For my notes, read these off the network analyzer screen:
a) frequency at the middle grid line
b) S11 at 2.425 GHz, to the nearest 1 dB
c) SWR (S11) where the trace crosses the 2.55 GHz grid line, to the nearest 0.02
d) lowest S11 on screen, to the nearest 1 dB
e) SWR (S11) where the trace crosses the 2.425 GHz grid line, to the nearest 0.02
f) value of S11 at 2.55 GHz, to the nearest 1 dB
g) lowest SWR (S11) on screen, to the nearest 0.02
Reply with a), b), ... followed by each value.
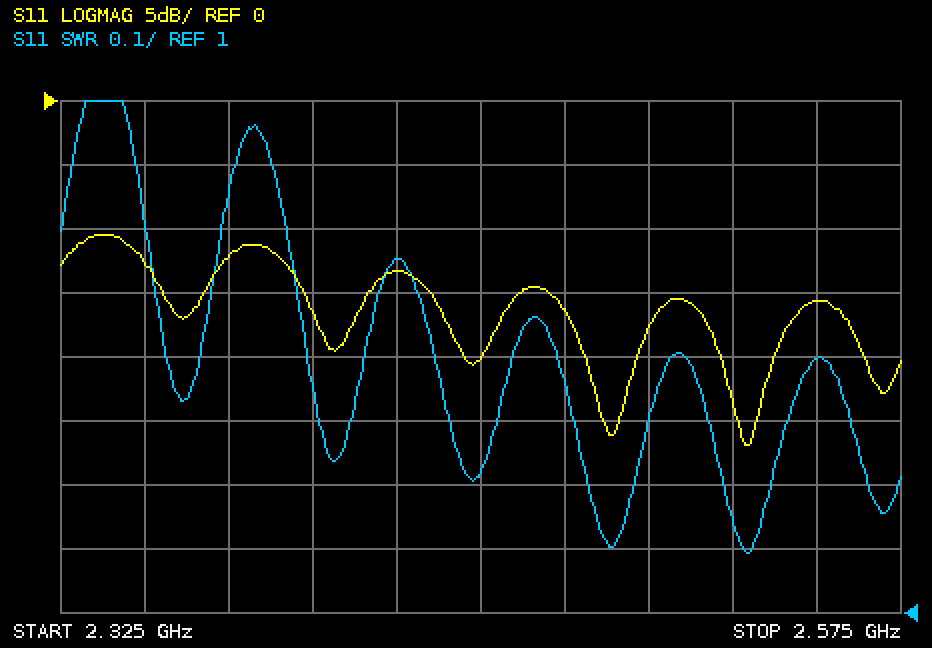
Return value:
a) 2.45 GHz
b) -13 dB
c) 1.40
d) -27 dB
e) 1.56
f) -16 dB
g) 1.10
